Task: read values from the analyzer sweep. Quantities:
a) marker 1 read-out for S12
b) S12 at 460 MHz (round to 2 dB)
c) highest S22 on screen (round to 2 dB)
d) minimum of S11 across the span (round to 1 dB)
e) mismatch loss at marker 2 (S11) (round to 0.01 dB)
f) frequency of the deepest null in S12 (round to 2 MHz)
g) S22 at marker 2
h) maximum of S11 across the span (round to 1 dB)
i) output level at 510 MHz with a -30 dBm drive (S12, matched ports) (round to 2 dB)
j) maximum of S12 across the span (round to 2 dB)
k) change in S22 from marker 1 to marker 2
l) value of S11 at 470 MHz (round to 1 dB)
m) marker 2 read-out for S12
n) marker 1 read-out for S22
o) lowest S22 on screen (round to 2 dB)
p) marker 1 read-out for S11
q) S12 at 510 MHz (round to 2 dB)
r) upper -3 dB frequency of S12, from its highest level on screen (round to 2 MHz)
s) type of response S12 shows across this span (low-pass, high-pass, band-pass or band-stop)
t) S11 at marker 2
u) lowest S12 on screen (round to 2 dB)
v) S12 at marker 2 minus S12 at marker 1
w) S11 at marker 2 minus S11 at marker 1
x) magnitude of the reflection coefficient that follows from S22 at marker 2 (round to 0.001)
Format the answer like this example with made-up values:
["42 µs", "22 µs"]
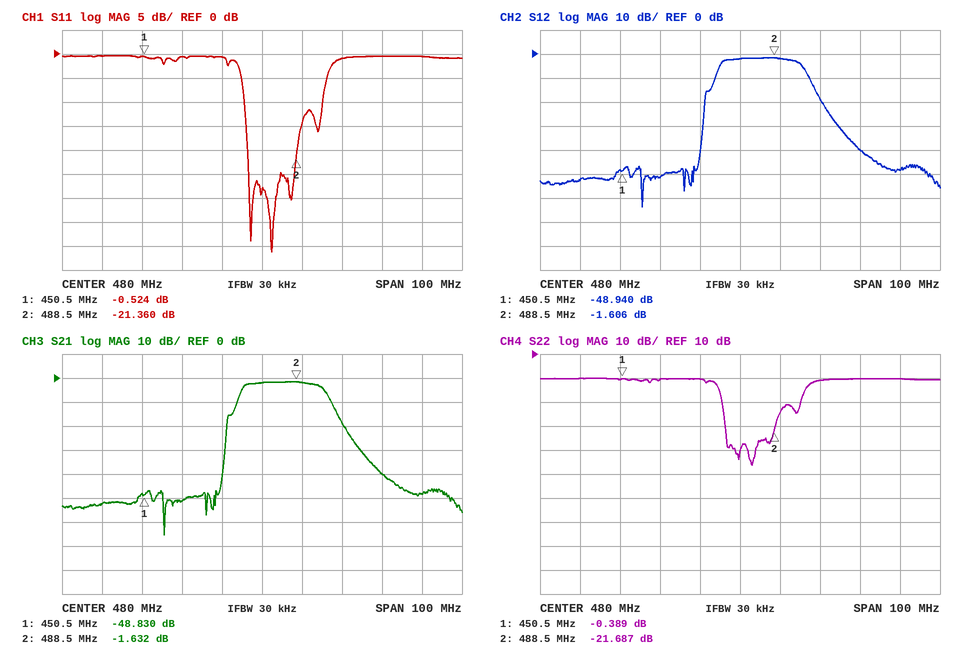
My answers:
["-48.940 dB", "-52 dB", "0 dB", "-41 dB", "0.03 dB", "456 MHz", "-21.687 dB", "0 dB", "-70 dBm", "-2 dB", "-21.298 dB", "-1 dB", "-1.606 dB", "-0.389 dB", "-36 dB", "-0.524 dB", "-40 dB", "496 MHz", "band-pass", "-21.360 dB", "-64 dB", "47.334 dB", "-20.836 dB", "0.082"]
